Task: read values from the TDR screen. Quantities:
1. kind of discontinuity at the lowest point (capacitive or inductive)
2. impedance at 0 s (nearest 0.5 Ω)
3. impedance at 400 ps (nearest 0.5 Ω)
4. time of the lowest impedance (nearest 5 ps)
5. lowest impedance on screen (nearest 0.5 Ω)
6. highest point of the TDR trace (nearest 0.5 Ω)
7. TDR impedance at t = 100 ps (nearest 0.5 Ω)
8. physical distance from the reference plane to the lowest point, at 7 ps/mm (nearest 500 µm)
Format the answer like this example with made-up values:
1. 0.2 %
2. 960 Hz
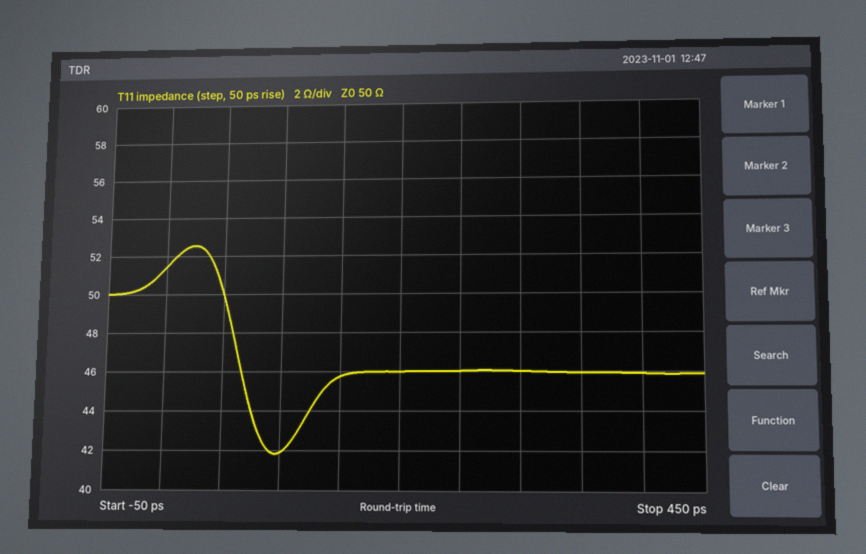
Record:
1. capacitive
2. 51.5 Ω
3. 46.0 Ω
4. 95 ps
5. 42.0 Ω
6. 52.5 Ω
7. 42.0 Ω
8. 7.0 mm
